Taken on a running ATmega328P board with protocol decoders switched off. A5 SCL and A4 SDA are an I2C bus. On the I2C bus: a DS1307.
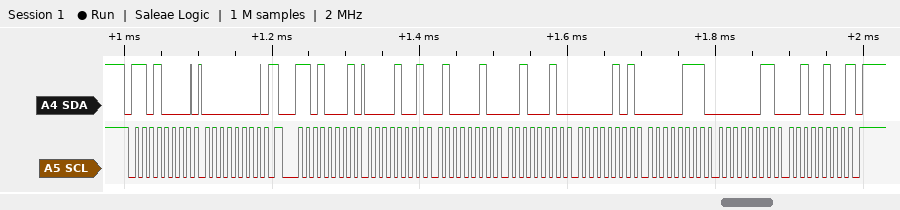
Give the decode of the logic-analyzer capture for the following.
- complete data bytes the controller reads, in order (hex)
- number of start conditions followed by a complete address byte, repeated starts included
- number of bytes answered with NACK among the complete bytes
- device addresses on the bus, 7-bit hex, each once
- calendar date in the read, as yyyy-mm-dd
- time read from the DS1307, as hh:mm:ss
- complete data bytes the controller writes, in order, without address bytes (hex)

09 42 22 05 07 03 24
2
1
0x68
2024-03-07
22:42:09
00
